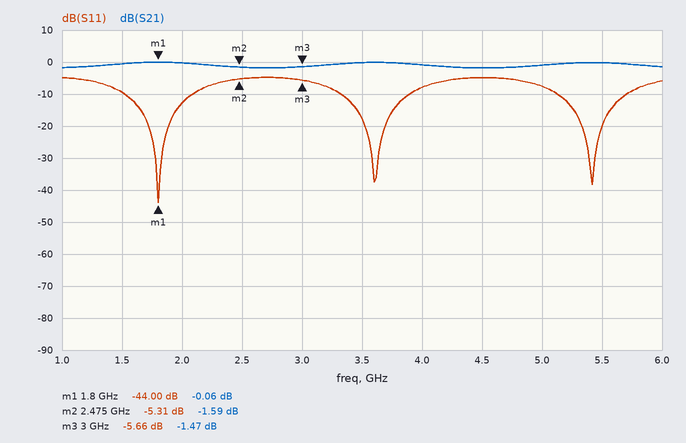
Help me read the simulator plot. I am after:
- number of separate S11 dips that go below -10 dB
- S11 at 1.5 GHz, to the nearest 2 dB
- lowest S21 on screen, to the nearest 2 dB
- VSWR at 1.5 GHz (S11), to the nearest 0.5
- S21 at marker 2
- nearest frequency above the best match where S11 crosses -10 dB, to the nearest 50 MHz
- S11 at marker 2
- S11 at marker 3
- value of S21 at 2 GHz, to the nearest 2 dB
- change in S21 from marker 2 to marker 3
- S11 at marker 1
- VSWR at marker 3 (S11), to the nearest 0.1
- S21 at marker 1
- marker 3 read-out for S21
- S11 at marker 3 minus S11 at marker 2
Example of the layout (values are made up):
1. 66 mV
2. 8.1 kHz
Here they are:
1. 3
2. -10 dB
3. -2 dB
4. 2.0
5. -1.59 dB
6. 2.10 GHz
7. -5.31 dB
8. -5.66 dB
9. 0 dB
10. 0.12 dB
11. -44.00 dB
12. 3.2
13. -0.06 dB
14. -1.47 dB
15. -0.35 dB
